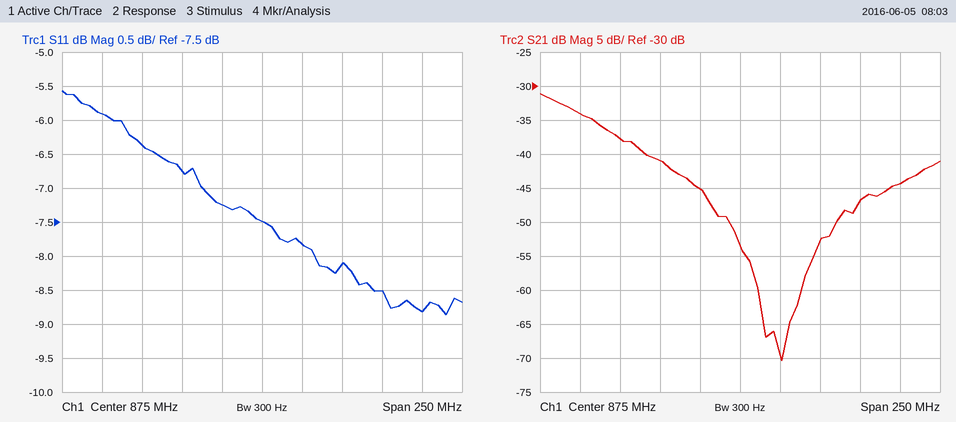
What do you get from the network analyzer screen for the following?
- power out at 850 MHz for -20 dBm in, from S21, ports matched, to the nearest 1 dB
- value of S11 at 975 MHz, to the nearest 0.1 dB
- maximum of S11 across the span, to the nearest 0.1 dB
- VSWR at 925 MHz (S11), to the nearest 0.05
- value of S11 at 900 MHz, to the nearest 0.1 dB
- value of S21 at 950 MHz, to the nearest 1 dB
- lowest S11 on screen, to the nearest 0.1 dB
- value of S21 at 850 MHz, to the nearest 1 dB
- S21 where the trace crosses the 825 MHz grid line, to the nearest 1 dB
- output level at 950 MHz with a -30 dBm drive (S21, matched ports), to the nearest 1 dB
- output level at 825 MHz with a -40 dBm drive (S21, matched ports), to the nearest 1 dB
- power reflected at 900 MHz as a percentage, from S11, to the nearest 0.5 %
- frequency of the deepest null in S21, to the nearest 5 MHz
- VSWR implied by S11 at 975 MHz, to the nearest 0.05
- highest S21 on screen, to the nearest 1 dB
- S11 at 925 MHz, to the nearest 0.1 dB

-65 dBm
-8.8 dB
-5.6 dB
2.30
-7.8 dB
-47 dB
-8.9 dB
-45 dB
-41 dB
-77 dBm
-81 dBm
16.5 %
900 MHz
2.15
-31 dB
-8.1 dB
